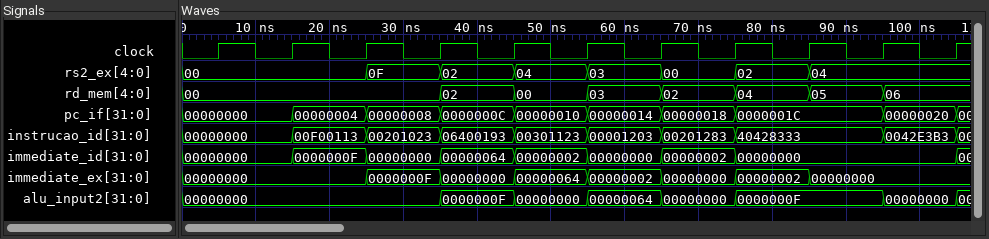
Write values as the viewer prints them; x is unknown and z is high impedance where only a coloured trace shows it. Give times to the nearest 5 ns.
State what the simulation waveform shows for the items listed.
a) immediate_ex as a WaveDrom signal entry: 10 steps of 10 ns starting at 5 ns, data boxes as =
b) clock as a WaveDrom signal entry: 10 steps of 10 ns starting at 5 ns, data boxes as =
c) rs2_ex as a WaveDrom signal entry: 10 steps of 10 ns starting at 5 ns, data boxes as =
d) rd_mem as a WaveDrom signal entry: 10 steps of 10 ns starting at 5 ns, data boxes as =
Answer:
{name: 'immediate_ex', wave: '=.=======.', data: '00000000 0000000F 00000000 00000064 00000002 00000000 00000002 00000000'}
{name: 'clock', wave: 'p.........'}
{name: 'rs2_ex', wave: '=.=======.', data: '00 0F 02 04 03 00 02 04'}
{name: 'rd_mem', wave: '=..=======', data: '00 02 00 03 02 04 05 06'}
